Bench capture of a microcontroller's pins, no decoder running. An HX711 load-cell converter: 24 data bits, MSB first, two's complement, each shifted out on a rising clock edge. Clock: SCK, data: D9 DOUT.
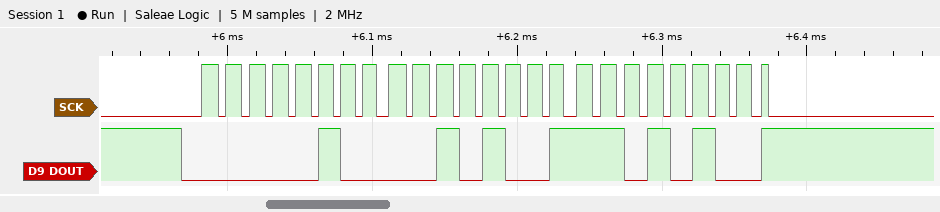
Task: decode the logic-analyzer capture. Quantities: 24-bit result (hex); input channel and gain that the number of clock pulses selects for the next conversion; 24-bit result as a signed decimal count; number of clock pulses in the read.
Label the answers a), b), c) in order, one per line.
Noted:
a) 0x0429D4
b) channel A, gain 128
c) 272852
d) 25
